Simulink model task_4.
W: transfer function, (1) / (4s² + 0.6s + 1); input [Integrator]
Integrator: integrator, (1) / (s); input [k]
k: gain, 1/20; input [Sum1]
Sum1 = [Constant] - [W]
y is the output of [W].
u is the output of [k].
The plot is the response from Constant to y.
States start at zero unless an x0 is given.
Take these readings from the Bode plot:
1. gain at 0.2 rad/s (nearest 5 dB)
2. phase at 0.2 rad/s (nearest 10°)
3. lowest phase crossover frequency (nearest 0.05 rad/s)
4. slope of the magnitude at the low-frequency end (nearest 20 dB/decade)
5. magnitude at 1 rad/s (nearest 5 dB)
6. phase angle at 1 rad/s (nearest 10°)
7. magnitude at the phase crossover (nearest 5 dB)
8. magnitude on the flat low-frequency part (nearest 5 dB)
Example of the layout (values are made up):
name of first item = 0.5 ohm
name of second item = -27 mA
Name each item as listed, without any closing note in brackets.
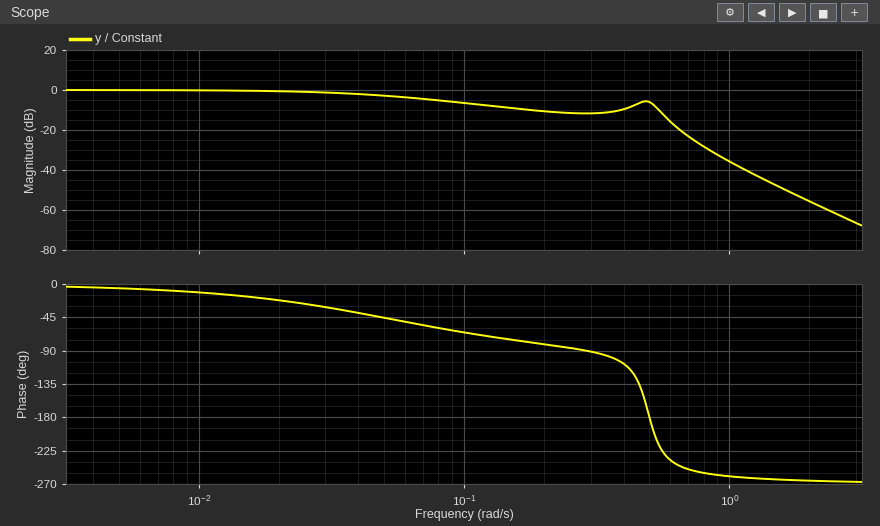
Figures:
gain at 0.2 rad/s = -10 dB
phase at 0.2 rad/s = -80°
lowest phase crossover frequency = 0.50 rad/s
slope of the magnitude at the low-frequency end = 0 dB/decade
magnitude at 1 rad/s = -35 dB
phase angle at 1 rad/s = -260°
magnitude at the phase crossover = -5 dB
magnitude on the flat low-frequency part = 0 dB
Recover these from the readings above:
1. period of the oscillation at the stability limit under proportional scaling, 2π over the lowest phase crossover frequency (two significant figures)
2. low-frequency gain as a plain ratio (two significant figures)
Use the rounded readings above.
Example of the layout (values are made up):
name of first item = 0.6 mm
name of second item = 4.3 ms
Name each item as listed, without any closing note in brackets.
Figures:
period of the oscillation at the stability limit under proportional scaling, 2π over the lowest phase crossover frequency = 13 s
low-frequency gain as a plain ratio = 1.0
